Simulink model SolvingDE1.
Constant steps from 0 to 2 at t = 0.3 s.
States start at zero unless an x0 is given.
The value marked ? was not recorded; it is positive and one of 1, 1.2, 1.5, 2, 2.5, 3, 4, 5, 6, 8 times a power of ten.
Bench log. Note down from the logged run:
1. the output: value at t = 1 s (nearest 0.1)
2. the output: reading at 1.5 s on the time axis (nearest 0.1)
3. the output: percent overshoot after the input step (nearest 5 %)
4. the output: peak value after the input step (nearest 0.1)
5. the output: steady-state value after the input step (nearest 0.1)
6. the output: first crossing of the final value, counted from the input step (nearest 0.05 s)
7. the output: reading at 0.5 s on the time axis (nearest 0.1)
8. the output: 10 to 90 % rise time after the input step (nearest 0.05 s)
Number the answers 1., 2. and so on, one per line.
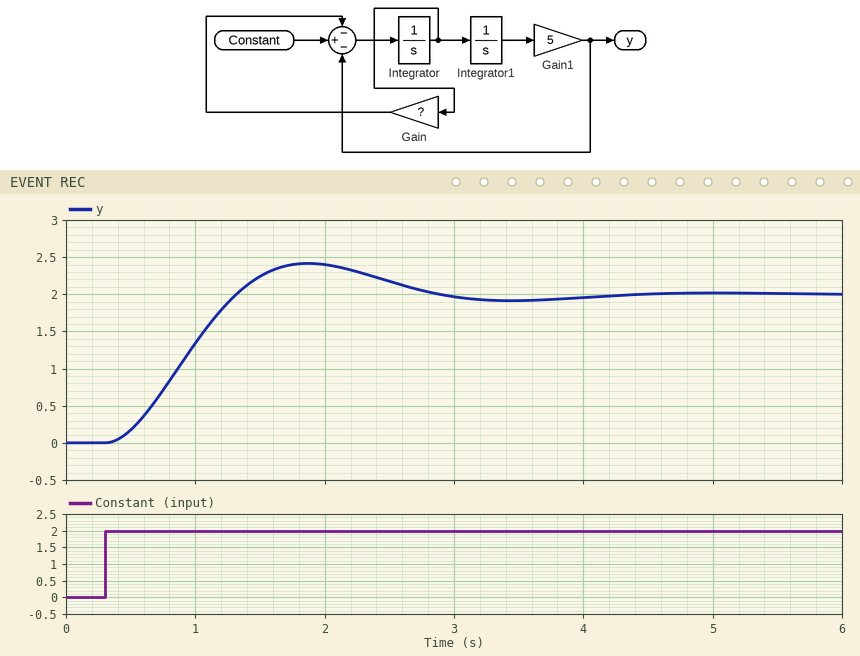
1. 1.3
2. 2.2
3. 20 %
4. 2.4
5. 2.0
6. 1.00 s
7. 0.2
8. 0.70 s
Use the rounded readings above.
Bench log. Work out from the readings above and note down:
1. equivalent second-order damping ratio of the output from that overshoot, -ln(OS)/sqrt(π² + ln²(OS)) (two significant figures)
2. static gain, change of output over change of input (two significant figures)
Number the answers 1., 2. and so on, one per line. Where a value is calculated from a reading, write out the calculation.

1. ln(0.2) = -1.609; 1.609 / sqrt(9.870 + 2.590) = 0.46
2. (2 - 0) / (2 - 0) = 1.0
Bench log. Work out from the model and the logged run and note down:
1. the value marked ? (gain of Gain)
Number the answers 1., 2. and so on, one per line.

1. 2
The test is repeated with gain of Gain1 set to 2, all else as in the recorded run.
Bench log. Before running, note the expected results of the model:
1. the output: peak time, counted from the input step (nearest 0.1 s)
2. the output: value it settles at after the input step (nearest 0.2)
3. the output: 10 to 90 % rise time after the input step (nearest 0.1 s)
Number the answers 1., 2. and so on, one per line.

1. 3.1 s
2. 2.0
3. 1.5 s
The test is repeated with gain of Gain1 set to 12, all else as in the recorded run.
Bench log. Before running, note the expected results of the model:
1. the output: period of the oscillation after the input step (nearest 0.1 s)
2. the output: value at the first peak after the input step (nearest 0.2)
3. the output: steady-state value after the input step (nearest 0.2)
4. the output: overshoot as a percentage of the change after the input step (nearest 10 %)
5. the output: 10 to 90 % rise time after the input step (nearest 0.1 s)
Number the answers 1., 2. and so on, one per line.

1. 1.9 s
2. 2.8
3. 2.0
4. 40 %
5. 0.4 s
